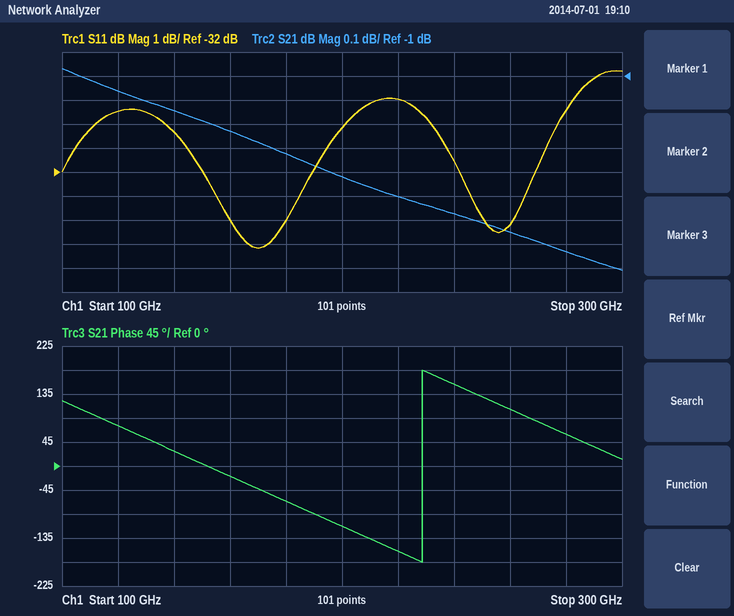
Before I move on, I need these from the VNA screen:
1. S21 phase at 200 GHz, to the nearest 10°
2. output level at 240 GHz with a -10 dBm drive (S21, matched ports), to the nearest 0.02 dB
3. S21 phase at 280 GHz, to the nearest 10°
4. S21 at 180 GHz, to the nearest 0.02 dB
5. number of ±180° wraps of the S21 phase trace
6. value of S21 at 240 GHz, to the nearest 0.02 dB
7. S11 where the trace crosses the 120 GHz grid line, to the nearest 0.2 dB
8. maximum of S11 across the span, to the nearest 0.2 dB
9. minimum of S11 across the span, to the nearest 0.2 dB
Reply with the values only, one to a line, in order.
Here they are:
-110°
-11.58 dBm
60°
-1.32 dB
1
-1.58 dB
-29.4 dB
-27.8 dB
-35.2 dB
